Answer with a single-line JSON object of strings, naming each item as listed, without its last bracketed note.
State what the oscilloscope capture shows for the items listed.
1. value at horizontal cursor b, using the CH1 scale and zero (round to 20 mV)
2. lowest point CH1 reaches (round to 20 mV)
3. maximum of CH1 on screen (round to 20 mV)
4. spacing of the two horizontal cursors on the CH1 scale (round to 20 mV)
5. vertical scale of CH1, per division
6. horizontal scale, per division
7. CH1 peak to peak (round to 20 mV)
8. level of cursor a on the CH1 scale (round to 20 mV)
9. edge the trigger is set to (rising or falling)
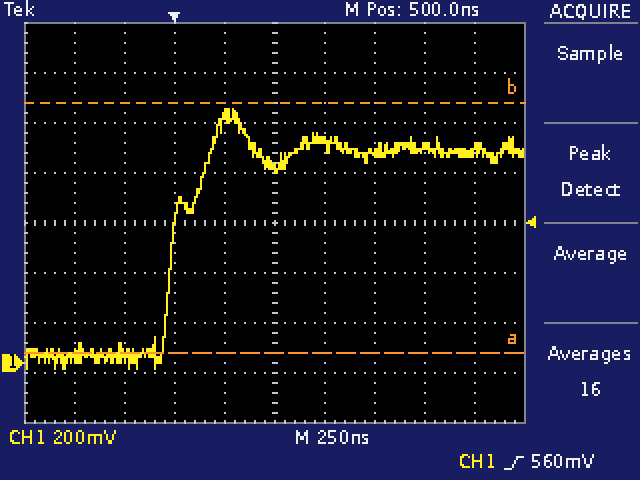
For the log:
{"value at horizontal cursor b, using the CH1 scale and zero": "1.04 V", "lowest point CH1 reaches": "-20 mV", "maximum of CH1 on screen": "1.02 V", "spacing of the two horizontal cursors on the CH1 scale": "1.00 V", "vertical scale of CH1, per division": "200 mV", "horizontal scale, per division": "250 ns", "CH1 peak to peak": "1.04 V", "level of cursor a on the CH1 scale": "40 mV", "edge the trigger is set to": "rising"}
